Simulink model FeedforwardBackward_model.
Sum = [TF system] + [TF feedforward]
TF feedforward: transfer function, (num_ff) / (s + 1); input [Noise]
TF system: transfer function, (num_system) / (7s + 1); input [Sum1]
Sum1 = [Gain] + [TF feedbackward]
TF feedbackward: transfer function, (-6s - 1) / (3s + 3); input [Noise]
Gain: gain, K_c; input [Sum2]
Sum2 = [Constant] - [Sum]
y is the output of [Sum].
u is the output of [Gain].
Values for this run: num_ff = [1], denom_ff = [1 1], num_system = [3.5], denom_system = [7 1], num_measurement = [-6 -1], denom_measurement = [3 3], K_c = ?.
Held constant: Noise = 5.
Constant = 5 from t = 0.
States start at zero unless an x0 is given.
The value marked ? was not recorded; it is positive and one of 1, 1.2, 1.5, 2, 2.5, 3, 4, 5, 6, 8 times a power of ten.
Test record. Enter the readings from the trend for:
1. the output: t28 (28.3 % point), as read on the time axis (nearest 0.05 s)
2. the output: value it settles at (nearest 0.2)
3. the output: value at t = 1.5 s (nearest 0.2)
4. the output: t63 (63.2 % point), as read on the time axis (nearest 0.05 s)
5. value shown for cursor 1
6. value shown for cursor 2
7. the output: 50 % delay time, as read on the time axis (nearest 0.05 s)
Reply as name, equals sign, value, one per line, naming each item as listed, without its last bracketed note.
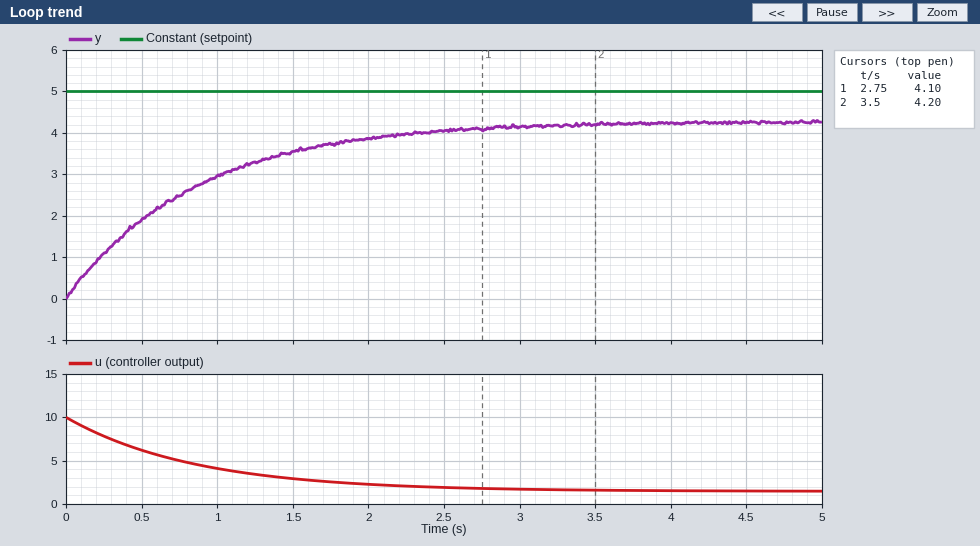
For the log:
the output: t28 (28.3 % point), as read on the time axis = 0.30 s
the output: value it settles at = 4.2
the output: value at t = 1.5 s = 3.6
the output: t63 (63.2 % point), as read on the time axis = 0.85 s
value shown for cursor 1 = 4.10
value shown for cursor 2 = 4.20
the output: 50 % delay time, as read on the time axis = 0.60 s
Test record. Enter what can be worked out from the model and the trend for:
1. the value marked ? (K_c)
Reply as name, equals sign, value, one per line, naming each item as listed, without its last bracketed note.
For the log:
the value marked ? = 2
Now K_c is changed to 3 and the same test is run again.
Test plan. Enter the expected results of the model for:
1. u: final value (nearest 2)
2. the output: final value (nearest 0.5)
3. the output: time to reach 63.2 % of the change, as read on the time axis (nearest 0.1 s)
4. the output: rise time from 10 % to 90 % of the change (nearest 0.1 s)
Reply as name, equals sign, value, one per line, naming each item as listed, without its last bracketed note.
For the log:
u: final value = 2
the output: final value = 4.5
the output: time to reach 63.2 % of the change, as read on the time axis = 0.6 s
the output: rise time from 10 % to 90 % of the change = 1.3 s
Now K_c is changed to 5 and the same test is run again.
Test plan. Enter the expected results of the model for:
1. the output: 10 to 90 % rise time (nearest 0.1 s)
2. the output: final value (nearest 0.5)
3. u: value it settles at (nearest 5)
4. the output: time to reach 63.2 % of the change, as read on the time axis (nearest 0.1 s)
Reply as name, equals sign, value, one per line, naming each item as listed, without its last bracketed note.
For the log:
the output: 10 to 90 % rise time = 0.8 s
the output: final value = 4.5
u: value it settles at = 0
the output: time to reach 63.2 % of the change, as read on the time axis = 0.4 s
